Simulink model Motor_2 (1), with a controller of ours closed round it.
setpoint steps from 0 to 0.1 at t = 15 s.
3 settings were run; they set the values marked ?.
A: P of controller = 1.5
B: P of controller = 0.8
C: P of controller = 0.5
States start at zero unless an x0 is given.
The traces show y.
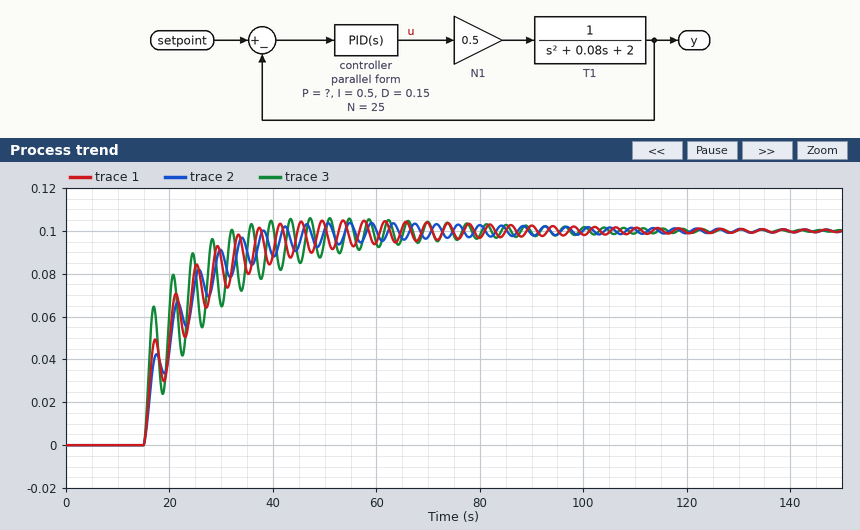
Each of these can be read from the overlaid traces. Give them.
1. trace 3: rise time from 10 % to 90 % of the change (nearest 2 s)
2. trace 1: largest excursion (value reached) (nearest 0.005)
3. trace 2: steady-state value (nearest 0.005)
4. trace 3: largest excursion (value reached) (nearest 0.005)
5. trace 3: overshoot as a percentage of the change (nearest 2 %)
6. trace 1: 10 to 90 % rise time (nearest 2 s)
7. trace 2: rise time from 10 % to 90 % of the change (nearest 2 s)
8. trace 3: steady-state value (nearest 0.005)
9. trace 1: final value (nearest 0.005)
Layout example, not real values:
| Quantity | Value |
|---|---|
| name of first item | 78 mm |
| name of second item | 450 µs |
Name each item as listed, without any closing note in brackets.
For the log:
| Quantity | Value |
|---|---|
| trace 3: rise time from 10 % to 90 % of the change | 12 s |
| trace 1: largest excursion (value reached) | 0.105 |
| trace 2: steady-state value | 0.100 |
| trace 3: largest excursion (value reached) | 0.105 |
| trace 3: overshoot as a percentage of the change | 6 % |
| trace 1: 10 to 90 % rise time | 14 s |
| trace 2: rise time from 10 % to 90 % of the change | 14 s |
| trace 3: steady-state value | 0.100 |
| trace 1: final value | 0.100 |
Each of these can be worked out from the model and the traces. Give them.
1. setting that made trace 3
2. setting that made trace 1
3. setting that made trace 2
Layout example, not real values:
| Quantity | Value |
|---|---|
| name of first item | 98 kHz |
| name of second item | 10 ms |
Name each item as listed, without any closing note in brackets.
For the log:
| Quantity | Value |
|---|---|
| setting that made trace 3 | A |
| setting that made trace 1 | B |
| setting that made trace 2 | C |
